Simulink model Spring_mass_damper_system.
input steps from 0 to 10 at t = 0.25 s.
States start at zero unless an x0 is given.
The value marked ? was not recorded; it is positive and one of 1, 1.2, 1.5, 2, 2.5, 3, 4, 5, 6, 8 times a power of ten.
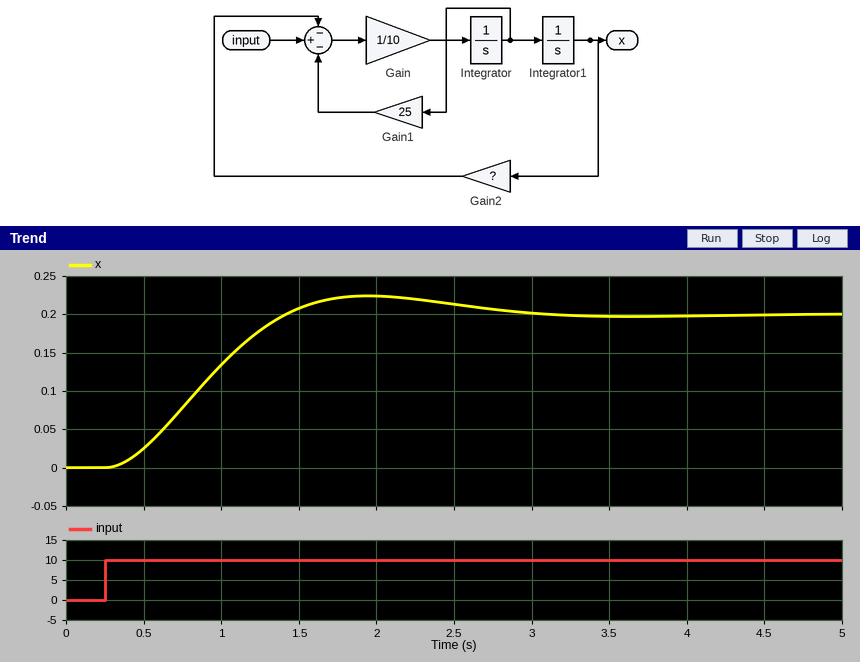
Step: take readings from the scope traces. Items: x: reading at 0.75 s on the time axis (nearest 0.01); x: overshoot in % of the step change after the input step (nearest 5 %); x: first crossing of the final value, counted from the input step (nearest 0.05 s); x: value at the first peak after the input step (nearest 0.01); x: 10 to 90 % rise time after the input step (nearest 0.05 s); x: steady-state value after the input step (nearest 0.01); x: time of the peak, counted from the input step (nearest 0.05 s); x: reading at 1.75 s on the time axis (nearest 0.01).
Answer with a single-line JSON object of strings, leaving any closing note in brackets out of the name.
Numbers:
{"x: reading at 0.75 s on the time axis": "0.08", "x: overshoot in % of the step change after the input step": "10 %", "x: first crossing of the final value, counted from the input step": "1.15 s", "x: value at the first peak after the input step": "0.22", "x: 10 to 90 % rise time after the input step": "0.80 s", "x: steady-state value after the input step": "0.20", "x: time of the peak, counted from the input step": "1.70 s", "x: reading at 1.75 s on the time axis": "0.22"}
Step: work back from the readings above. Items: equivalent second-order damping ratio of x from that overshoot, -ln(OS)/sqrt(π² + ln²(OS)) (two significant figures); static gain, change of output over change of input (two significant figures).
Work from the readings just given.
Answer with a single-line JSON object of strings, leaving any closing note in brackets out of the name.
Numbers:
{"equivalent second-order damping ratio of x from that overshoot, -ln(OS)/sqrt(π² + ln²(OS))": "0.59", "static gain, change of output over change of input": "0.020"}
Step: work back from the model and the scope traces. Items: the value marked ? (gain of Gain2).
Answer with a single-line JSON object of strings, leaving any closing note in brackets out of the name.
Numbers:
{"the value marked ?": "50"}
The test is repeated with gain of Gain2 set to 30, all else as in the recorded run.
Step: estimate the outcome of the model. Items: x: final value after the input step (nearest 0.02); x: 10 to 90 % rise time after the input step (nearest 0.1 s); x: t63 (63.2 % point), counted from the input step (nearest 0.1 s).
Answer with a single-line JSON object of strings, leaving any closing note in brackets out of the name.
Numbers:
{"x: final value after the input step": "0.34", "x: 10 to 90 % rise time after the input step": "1.3 s", "x: t63 (63.2 % point), counted from the input step": "1.0 s"}
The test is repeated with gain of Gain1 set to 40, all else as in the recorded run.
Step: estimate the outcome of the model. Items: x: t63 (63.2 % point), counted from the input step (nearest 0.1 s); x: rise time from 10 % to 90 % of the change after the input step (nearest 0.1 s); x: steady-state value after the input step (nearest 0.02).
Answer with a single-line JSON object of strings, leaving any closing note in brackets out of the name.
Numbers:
{"x: t63 (63.2 % point), counted from the input step": "0.9 s", "x: rise time from 10 % to 90 % of the change after the input step": "1.3 s", "x: steady-state value after the input step": "0.20"}
